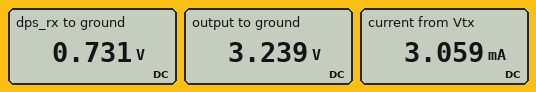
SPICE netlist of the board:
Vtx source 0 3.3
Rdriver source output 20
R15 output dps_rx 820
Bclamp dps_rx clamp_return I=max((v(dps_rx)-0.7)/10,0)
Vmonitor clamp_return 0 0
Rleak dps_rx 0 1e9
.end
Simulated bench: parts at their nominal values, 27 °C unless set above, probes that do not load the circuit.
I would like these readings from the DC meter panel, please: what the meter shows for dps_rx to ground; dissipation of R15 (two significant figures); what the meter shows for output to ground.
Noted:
0.731 V
7.7 mW
3.239 V
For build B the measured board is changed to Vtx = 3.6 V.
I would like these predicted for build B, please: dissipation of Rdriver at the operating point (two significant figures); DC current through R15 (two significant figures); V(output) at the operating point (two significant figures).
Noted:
230 µW
3.4 mA
3.5 V
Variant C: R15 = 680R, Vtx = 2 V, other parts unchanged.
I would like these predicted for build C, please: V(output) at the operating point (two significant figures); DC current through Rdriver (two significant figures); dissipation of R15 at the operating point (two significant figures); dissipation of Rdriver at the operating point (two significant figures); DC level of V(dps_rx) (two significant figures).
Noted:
2.0 V
1.8 mA
2.3 mW
67 µW
720 mV
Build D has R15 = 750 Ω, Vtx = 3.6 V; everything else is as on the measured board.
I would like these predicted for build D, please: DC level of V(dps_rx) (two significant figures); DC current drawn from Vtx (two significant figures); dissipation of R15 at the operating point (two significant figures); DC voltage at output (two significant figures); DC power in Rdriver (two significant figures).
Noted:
740 mV
3.7 mA
10 mW
3.5 V
280 µW
